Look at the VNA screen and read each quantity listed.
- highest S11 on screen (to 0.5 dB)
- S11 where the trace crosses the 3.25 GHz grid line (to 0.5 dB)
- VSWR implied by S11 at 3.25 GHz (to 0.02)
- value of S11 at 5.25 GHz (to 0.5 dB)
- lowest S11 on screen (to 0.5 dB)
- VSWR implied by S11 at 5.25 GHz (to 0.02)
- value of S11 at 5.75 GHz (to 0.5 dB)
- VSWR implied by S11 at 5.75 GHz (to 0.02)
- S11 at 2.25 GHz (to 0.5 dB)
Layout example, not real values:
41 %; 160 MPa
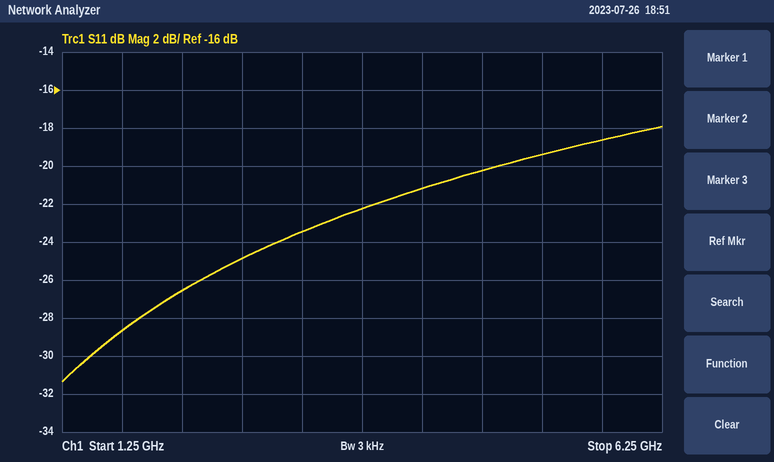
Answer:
-18.0 dB; -23.5 dB; 1.14; -19.5 dB; -31.5 dB; 1.24; -18.5 dB; 1.26; -26.5 dB
